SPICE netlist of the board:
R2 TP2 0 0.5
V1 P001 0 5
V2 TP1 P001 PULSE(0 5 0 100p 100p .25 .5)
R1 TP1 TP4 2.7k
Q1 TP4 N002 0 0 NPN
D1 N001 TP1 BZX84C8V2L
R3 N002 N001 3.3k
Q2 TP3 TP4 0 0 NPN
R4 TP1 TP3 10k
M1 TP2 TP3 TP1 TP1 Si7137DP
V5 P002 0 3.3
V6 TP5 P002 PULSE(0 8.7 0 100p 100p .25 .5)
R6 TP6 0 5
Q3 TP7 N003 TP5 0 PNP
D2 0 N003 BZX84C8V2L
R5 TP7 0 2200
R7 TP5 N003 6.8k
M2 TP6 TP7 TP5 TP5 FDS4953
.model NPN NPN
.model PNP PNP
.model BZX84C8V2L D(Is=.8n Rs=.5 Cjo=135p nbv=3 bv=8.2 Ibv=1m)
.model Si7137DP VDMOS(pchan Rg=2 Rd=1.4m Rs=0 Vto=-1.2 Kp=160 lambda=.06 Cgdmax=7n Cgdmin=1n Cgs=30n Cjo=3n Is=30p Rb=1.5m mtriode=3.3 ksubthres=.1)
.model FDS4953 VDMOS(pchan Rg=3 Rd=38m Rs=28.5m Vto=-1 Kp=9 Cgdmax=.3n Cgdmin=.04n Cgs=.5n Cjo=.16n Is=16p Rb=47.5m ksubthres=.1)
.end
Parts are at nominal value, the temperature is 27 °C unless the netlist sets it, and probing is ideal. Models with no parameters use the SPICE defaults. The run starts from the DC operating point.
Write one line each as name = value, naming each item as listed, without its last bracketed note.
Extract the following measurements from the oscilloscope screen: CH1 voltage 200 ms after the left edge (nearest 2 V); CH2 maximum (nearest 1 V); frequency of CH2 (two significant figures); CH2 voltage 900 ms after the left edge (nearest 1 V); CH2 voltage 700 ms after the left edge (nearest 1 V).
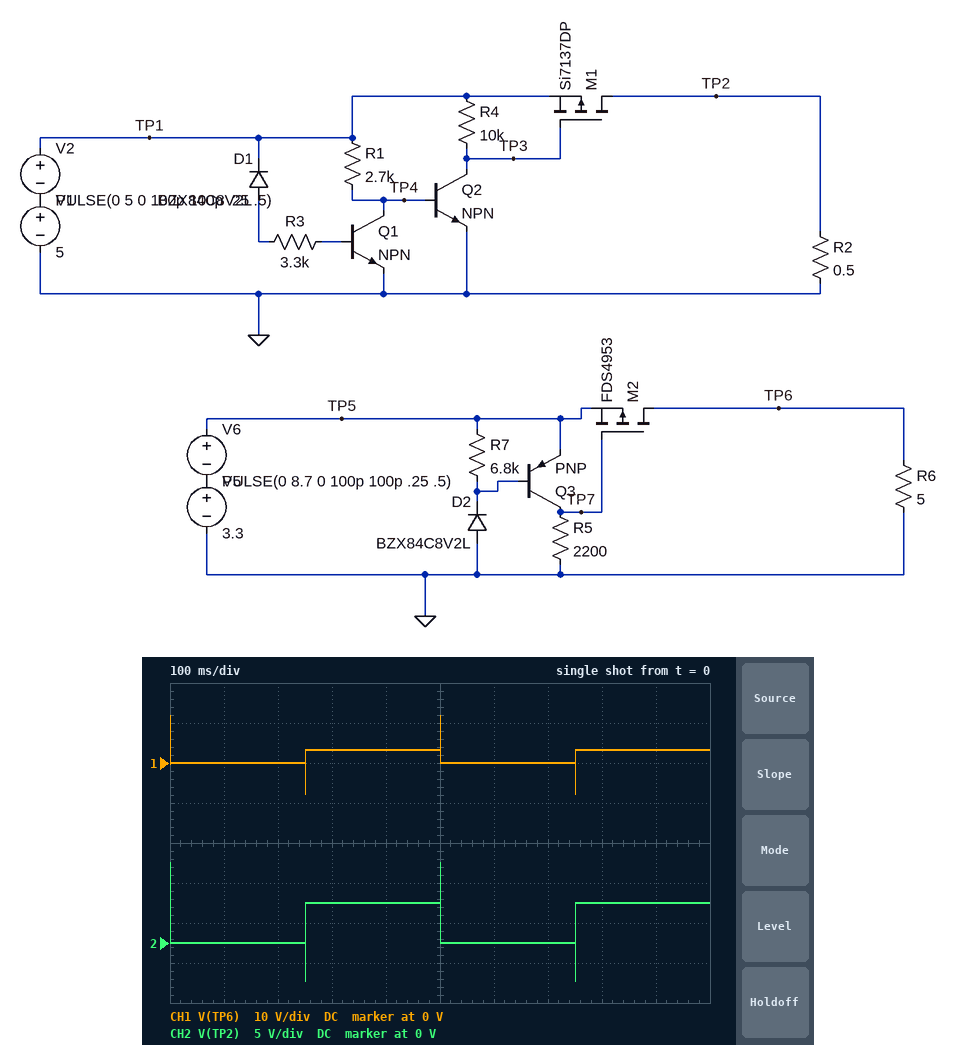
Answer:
CH1 voltage 200 ms after the left edge = 0 V
CH2 maximum = 10 V
frequency of CH2 = 2.0 Hz
CH2 voltage 900 ms after the left edge = 5 V
CH2 voltage 700 ms after the left edge = 0 V
